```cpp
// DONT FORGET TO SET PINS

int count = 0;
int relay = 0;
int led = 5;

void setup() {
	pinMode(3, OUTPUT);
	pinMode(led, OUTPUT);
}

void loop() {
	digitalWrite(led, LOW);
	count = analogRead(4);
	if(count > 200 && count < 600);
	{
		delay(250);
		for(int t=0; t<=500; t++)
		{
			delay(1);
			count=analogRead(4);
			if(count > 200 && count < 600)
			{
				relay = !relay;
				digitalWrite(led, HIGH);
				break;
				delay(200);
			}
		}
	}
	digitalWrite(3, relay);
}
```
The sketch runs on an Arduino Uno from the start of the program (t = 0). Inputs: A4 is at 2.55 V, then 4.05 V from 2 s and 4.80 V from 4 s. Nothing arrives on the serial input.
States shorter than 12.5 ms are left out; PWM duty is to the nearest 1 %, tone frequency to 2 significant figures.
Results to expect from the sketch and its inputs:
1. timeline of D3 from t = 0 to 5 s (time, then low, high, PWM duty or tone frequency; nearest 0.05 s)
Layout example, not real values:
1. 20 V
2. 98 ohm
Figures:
1. 0 s low; 0.25 s high; 0.5 s low; 0.75 s high; 1 s low; 1.25 s high; 1.5 s low; 1.75 s high
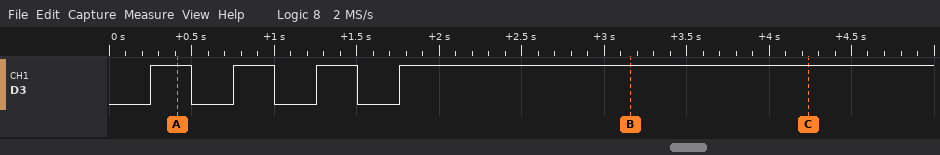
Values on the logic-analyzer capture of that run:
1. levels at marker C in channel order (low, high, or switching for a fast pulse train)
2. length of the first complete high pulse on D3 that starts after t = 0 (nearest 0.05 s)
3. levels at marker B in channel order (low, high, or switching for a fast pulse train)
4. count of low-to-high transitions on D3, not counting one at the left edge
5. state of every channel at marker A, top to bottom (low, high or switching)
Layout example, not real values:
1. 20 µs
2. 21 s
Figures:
1. D3 high
2. 0.25 s
3. D3 high
4. 4
5. D3 high
